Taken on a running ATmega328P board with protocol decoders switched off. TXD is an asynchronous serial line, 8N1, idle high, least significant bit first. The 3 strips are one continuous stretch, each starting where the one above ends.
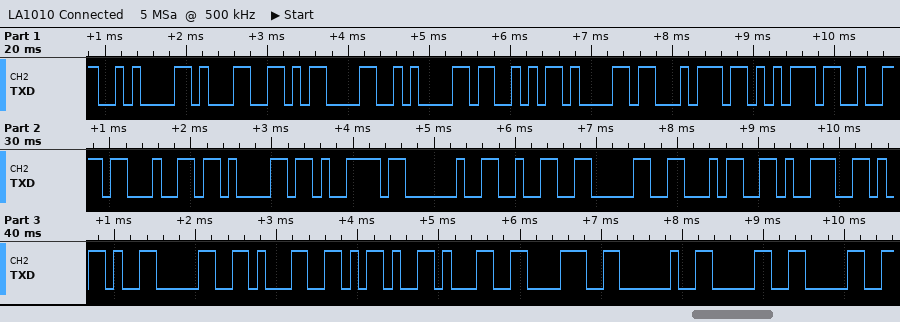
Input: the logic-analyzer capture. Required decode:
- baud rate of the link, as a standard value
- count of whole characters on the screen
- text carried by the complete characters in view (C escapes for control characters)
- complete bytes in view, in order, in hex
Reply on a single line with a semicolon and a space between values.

9600 baud; 26; "\n1\r\nSaturday 2049-01-18 00"; 0A 31 0D 0A 53 61 74 75 72 64 61 79 20 32 30 34 39 2D 30 31 2D 31 38 20 30 30
